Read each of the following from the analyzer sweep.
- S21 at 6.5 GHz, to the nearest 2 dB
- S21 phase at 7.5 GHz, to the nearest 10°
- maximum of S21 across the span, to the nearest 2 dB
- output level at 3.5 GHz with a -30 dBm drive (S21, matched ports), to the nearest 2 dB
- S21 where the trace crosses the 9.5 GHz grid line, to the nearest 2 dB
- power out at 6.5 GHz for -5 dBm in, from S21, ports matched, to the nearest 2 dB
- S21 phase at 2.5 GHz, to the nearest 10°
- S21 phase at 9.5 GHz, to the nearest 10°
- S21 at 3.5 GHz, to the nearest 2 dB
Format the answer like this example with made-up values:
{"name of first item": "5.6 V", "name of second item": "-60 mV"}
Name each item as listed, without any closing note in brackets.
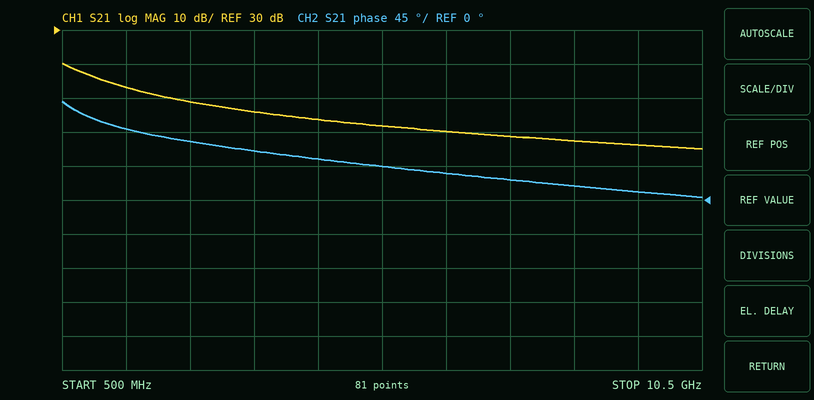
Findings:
{"S21 at 6.5 GHz, to the nearest 2 dB": "0 dB", "S21 phase at 7.5 GHz, to the nearest 10°": "30°", "maximum of S21 across the span, to the nearest 2 dB": "20 dB", "output level at 3.5 GHz with a -30 dBm drive (S21, matched ports), to the nearest 2 dB": "-24 dBm", "S21 where the trace crosses the 9.5 GHz grid line, to the nearest 2 dB": "-4 dB", "power out at 6.5 GHz for -5 dBm in, from S21, ports matched, to the nearest 2 dB": "-4 dBm", "S21 phase at 2.5 GHz, to the nearest 10°": "80°", "S21 phase at 9.5 GHz, to the nearest 10°": "10°", "S21 at 3.5 GHz, to the nearest 2 dB": "6 dB"}
